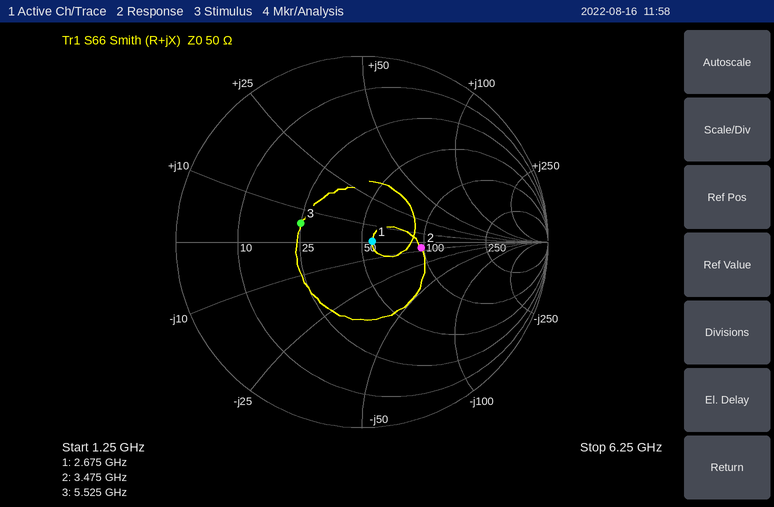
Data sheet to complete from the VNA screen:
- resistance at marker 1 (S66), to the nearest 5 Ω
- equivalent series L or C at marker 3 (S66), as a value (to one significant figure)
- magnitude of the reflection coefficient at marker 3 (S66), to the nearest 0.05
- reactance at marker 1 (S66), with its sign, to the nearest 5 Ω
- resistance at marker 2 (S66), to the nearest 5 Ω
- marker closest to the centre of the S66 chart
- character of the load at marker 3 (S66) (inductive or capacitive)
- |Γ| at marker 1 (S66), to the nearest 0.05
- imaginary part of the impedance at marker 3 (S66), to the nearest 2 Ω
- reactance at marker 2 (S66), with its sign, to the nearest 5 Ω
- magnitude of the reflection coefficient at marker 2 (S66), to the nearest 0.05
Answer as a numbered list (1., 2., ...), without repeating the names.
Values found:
1. 55 Ω
2. 200 pH
3. 0.35
4. 0 Ω
5. 95 Ω
6. marker 1
7. inductive
8. 0.05
9. +6 Ω
10. -5 Ω
11. 0.30
